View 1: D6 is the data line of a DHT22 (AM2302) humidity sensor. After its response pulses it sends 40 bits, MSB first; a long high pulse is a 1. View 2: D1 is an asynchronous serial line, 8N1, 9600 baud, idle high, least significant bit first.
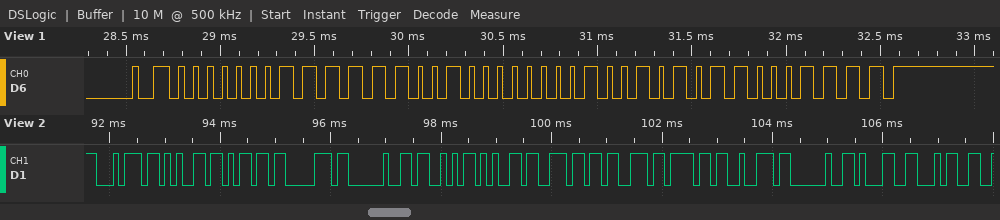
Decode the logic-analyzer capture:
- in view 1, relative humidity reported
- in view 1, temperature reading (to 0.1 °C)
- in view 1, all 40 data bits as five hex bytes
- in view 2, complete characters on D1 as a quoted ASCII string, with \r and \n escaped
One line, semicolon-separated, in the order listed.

50.5 %; 14.9 °C; 01 F9 00 95 8F; "temp Sensor 14"
